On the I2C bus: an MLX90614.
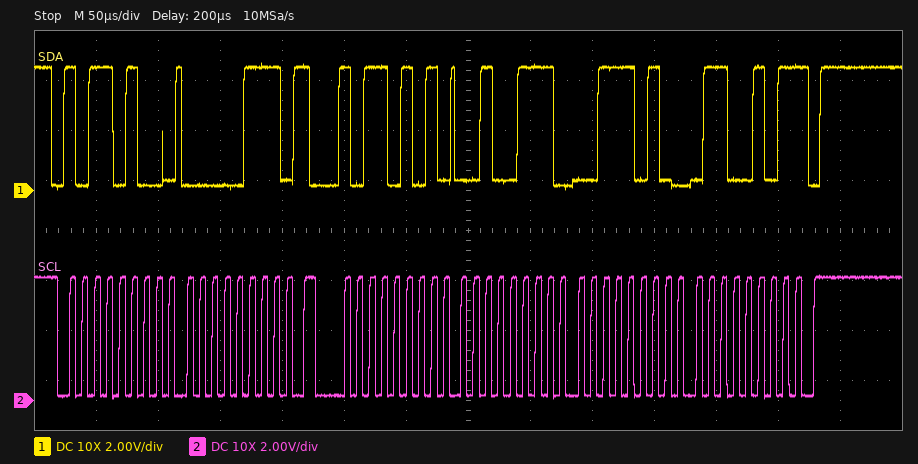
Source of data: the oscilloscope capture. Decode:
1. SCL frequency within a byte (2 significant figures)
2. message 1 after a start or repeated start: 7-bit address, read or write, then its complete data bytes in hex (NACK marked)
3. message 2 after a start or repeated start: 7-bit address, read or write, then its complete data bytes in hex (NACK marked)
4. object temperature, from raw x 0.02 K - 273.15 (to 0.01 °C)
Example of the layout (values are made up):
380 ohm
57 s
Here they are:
100 kHz
0x5A write: 07
0x5A read: 27 3A 65 NACK
24.59 °C
